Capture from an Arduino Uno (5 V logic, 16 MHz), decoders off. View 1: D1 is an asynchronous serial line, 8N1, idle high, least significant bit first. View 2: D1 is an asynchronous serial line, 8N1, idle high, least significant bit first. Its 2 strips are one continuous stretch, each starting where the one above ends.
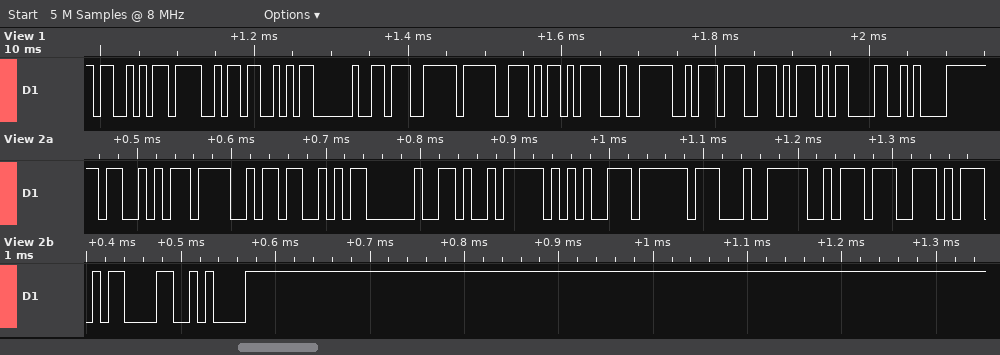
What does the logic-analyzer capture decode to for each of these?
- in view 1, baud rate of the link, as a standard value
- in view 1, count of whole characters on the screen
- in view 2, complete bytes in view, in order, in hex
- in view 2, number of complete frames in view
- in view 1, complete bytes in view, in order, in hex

115200 baud
12
0x53 0x4F 0x53 0x20 0xE9 0x95 0xBF 0xE4 0xBA 0xAE 0x0D 0x0A
12
53 4F 53 20 E7 9F AD E4 BA AE 0D 0A
